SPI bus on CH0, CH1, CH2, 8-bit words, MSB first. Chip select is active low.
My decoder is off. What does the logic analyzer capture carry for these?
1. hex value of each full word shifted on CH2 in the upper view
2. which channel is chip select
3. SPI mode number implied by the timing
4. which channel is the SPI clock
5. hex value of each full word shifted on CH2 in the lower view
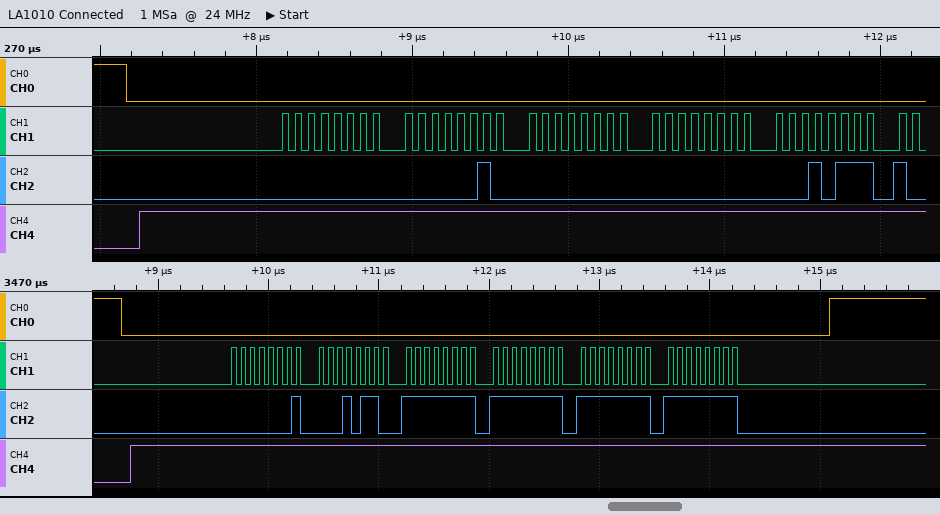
00, 02, 00, 00, 17
CH0
0
CH1
01, 16, FF, FF, FF, FF
